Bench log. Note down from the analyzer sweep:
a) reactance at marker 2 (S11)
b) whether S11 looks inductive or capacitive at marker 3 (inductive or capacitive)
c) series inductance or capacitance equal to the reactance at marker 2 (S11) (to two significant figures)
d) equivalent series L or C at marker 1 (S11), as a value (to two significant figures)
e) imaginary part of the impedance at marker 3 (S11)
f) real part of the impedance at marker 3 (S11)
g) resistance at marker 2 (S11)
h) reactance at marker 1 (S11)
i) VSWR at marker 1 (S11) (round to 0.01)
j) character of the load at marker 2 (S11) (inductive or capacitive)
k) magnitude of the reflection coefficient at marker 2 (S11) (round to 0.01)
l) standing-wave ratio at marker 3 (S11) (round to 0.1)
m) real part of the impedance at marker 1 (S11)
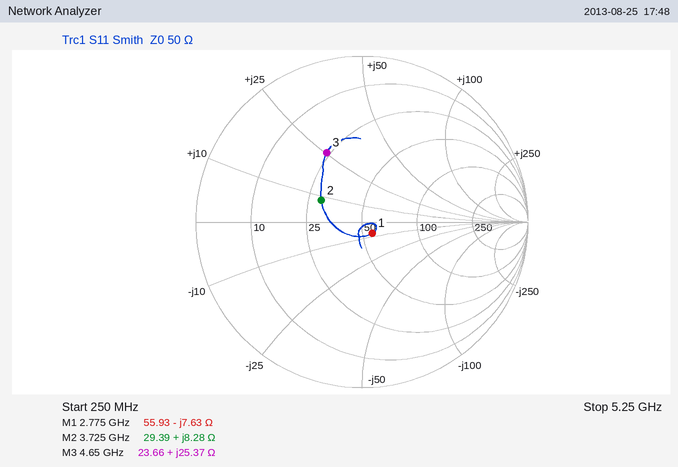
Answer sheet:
+8.28 Ω
inductive
350 pH
7.5 pF
+25.37 Ω
23.66 Ω
29.39 Ω
-7.63 Ω
1.20
inductive
0.28
2.8
55.93 Ω
